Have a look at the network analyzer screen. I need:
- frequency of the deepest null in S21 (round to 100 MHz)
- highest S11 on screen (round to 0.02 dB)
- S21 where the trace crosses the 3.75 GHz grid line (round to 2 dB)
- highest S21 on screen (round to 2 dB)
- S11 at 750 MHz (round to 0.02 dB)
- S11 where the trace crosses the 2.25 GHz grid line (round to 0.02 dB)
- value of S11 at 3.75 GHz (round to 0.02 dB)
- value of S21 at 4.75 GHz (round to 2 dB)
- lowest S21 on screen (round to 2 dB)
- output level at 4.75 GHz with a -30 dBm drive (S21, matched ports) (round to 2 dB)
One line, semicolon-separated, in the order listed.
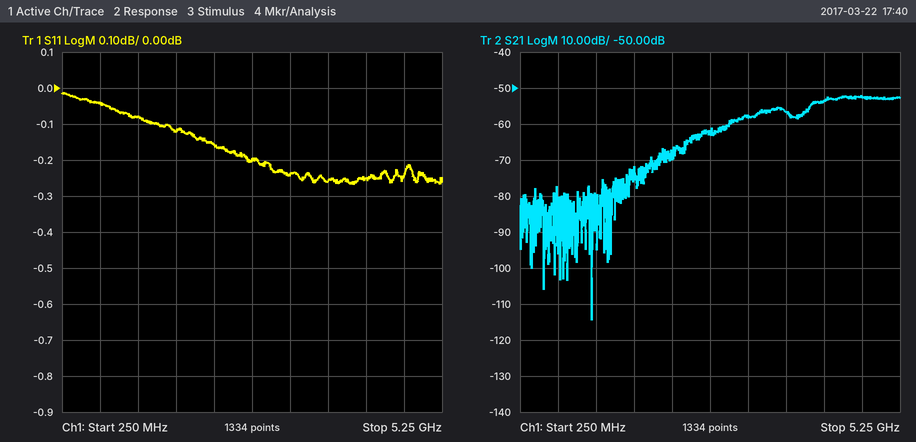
1.2 GHz; -0.02 dB; -56 dB; -52 dB; -0.04 dB; -0.16 dB; -0.26 dB; -52 dB; -114 dB; -82 dBm
